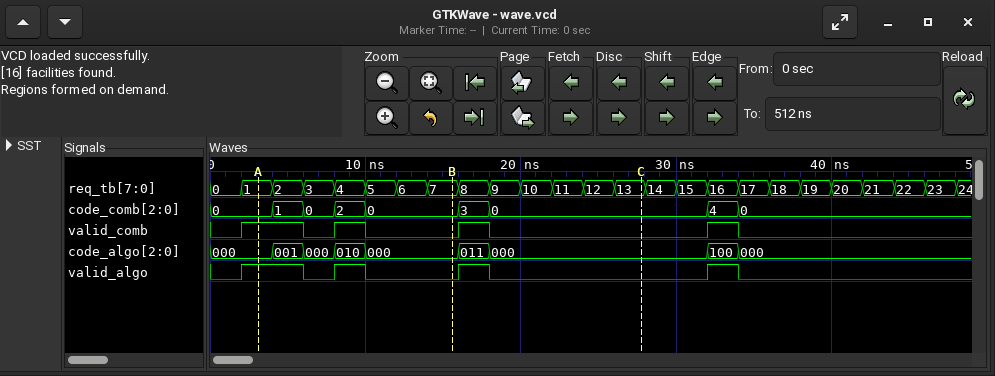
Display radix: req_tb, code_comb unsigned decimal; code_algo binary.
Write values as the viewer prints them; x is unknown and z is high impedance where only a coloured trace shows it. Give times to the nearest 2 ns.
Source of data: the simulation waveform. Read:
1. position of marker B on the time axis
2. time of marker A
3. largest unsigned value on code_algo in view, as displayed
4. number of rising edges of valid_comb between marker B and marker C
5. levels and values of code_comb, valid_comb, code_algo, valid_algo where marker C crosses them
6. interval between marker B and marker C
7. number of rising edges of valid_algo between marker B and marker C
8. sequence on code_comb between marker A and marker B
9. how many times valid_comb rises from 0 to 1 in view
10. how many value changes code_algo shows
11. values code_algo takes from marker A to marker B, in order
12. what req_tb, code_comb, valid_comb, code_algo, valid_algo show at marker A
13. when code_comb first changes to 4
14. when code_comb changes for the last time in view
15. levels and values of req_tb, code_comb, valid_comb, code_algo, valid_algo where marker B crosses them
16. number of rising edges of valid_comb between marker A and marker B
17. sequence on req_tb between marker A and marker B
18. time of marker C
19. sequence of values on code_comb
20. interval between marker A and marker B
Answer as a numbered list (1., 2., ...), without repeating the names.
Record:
1. 16 ns
2. 4 ns
3. 100
4. 1
5. code_comb=0, valid_comb=0, code_algo=000, valid_algo=0
6. 12 ns
7. 1
8. 0, 1, 0, 2, 0
9. 4
10. 8
11. 000, 001, 000, 010, 000
12. req_tb=1, code_comb=0, valid_comb=1, code_algo=000, valid_algo=1
13. 32 ns
14. 34 ns
15. req_tb=7, code_comb=0, valid_comb=0, code_algo=000, valid_algo=0
16. 1
17. 1, 2, 3, 4, 5, 6, 7
18. 28 ns
19. 0, 1, 0, 2, 0, 3, 0, 4, 0
20. 12 ns
